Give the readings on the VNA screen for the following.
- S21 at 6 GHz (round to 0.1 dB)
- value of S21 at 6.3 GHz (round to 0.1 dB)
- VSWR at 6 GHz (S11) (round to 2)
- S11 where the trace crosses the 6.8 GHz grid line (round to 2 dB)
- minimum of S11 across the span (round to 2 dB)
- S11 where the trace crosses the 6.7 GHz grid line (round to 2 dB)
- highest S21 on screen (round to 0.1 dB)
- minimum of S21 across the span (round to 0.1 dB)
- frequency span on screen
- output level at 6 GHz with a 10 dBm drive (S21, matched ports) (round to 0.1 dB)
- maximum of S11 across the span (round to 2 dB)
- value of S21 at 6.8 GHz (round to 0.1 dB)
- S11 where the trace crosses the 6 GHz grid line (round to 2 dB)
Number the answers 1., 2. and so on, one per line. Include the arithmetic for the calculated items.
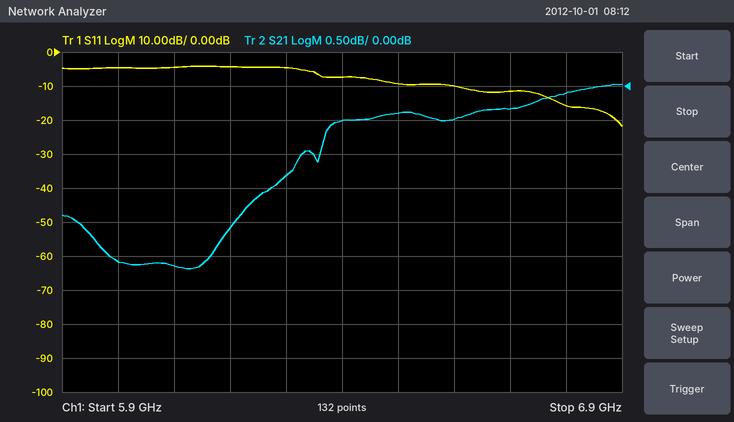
1. -2.6 dB
2. -1.3 dB
3. |Γ| = 10^(-4/20) = 0.6310; VSWR = (1 + 0.6310)/(1 − 0.6310) ≈ 4
4. -16 dB
5. -22 dB
6. -12 dB
7. 0.0 dB
8. -2.7 dB
9. 1 GHz
10. 10 dBm + (-2.6 dB) = 7.4 dBm
11. -4 dB
12. -0.1 dB
13. -4 dB
